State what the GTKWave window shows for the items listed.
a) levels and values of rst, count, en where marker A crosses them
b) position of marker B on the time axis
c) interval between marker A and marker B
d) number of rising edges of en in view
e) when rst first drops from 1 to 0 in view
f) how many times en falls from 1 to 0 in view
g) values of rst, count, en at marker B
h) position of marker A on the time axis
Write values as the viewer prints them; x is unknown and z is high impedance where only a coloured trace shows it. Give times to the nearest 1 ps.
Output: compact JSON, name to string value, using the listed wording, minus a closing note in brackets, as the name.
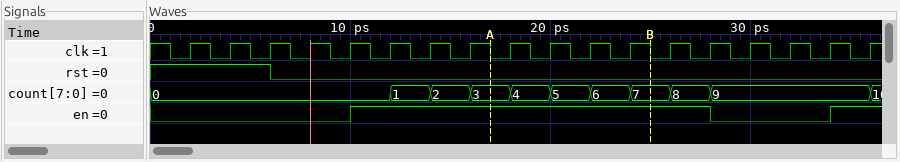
{"levels and values of rst, count, en where marker A crosses them": "rst=0, count=3, en=1", "position of marker B on the time axis": "25 ps", "interval between marker A and marker B": "8 ps", "number of rising edges of en in view": "2", "when rst first drops from 1 to 0 in view": "6 ps", "how many times en falls from 1 to 0 in view": "1", "values of rst, count, en at marker B": "rst=0, count=7, en=1", "position of marker A on the time axis": "17 ps"}
